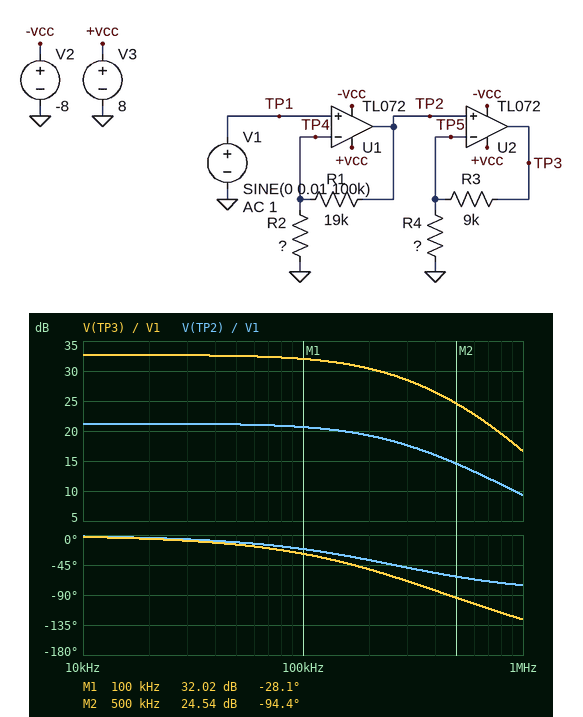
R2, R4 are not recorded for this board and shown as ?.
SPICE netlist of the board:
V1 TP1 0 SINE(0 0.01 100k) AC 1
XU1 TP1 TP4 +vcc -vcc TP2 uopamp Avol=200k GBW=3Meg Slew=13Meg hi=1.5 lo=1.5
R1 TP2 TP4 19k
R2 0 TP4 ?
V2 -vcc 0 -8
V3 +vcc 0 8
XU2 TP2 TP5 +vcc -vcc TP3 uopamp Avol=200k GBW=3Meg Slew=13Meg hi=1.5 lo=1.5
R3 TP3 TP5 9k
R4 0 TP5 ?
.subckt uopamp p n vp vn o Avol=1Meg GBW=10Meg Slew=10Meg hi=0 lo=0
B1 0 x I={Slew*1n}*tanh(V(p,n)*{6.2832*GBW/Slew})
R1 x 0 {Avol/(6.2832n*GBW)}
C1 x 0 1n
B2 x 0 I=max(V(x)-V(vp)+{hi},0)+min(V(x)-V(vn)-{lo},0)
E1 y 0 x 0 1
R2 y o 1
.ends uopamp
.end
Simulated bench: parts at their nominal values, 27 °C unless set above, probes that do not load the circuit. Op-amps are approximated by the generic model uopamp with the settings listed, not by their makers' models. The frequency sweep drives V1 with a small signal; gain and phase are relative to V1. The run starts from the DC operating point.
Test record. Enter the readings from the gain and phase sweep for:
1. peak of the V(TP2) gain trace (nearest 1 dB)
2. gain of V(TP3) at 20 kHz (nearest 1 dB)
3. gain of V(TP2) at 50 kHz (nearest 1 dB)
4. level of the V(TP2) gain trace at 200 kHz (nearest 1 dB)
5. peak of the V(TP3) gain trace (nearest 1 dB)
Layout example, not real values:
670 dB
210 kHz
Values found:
21 dB
33 dB
21 dB
19 dB
33 dB
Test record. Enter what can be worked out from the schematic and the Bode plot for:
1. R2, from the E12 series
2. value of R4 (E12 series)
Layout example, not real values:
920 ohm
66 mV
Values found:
1.8 kΩ
3.3 kΩ
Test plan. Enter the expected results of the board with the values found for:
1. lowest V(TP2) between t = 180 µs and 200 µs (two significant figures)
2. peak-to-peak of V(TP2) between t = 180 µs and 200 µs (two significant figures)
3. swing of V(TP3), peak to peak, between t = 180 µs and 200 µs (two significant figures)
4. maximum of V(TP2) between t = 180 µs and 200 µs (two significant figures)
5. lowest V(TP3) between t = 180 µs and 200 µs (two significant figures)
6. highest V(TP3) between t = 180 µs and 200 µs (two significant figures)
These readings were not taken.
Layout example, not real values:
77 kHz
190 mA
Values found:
-110 mV
220 mV
800 mV
110 mV
-400 mV
400 mV
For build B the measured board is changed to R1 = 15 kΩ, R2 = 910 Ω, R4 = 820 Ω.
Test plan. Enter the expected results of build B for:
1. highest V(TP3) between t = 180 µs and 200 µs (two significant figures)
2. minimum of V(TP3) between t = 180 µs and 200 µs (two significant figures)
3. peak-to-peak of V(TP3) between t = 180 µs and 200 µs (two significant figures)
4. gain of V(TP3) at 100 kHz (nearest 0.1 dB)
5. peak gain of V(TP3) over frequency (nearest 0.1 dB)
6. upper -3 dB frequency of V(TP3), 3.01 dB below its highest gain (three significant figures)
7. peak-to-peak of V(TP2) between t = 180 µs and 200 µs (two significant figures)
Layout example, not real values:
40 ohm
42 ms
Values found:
1.7 V
-1.7 V
3.4 V
44.5 dB
46.4 dB
130 kHz
300 mV
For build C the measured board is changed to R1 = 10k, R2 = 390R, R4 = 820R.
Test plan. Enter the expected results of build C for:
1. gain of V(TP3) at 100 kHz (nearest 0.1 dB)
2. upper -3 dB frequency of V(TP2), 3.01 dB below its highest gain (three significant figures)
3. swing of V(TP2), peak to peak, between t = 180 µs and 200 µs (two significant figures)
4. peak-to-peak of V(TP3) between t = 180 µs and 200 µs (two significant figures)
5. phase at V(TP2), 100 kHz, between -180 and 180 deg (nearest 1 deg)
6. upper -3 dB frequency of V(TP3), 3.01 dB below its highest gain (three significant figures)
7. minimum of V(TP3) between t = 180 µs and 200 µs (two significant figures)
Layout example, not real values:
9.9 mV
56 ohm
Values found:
46.9 dB
113 kHz
400 mV
4.4 V
-42 deg
96.9 kHz
-2.2 V
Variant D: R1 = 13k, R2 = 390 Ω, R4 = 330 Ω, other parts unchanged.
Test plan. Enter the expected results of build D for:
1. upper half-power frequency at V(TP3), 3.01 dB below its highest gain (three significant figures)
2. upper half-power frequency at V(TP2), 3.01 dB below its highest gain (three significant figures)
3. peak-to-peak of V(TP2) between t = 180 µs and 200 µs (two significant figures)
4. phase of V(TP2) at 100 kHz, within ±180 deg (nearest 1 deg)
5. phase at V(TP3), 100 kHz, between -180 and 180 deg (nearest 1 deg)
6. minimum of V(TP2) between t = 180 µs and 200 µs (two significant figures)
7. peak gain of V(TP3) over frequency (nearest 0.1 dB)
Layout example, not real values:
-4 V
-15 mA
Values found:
61.6 kHz
87.4 kHz
450 mV
-49 deg
-92 deg
-230 mV
59.7 dB
